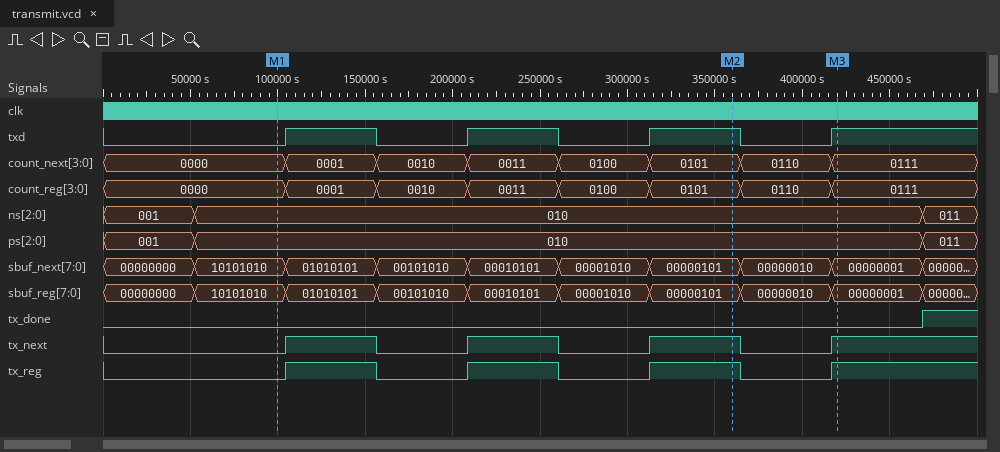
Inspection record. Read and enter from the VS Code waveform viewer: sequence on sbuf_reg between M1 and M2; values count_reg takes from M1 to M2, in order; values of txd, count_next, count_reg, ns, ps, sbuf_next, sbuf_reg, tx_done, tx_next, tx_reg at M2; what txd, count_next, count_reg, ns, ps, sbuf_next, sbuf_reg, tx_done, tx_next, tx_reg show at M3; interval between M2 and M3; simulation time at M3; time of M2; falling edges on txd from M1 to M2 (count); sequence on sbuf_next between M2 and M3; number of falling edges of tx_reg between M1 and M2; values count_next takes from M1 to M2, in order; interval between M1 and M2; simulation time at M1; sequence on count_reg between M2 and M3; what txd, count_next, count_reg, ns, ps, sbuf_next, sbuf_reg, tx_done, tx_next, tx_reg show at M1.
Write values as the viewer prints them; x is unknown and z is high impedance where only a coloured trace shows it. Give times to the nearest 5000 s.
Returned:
10101010, 01010101, 00101010, 00010101, 00001010, 00000101
0000, 0001, 0010, 0011, 0100, 0101
txd=1, count_next=0101, count_reg=0101, ns=010, ps=010, sbuf_next=00000101, sbuf_reg=00000101, tx_done=0, tx_next=1, tx_reg=1
txd=1, count_next=0111, count_reg=0111, ns=010, ps=010, sbuf_next=00000001, sbuf_reg=00000001, tx_done=0, tx_next=1, tx_reg=1
60000 s
420000 s
360000 s
2
00000101, 00000010, 00000001
2
0000, 0001, 0010, 0011, 0100, 0101
260000 s
100000 s
0101, 0110, 0111
txd=0, count_next=0000, count_reg=0000, ns=010, ps=010, sbuf_next=10101010, sbuf_reg=10101010, tx_done=0, tx_next=0, tx_reg=0
